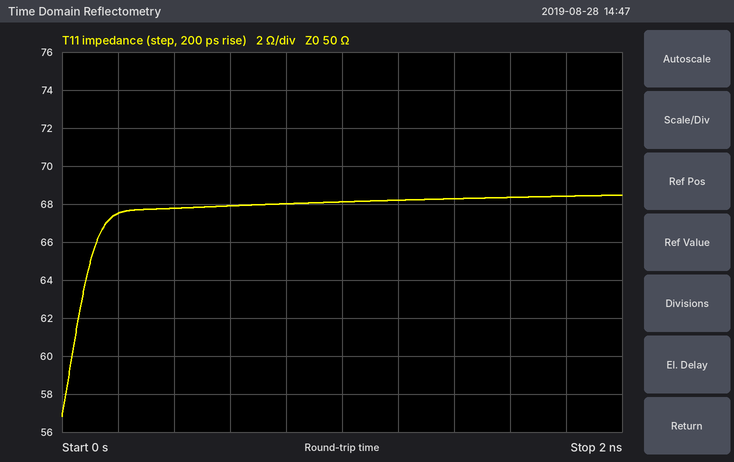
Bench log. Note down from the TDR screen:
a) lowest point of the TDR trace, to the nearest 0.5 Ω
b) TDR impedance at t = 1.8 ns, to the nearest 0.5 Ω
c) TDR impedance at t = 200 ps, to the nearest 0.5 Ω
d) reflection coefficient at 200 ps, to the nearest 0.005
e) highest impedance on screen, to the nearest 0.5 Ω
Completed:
57.0 Ω
68.5 Ω
67.5 Ω
+0.150
68.5 Ω
